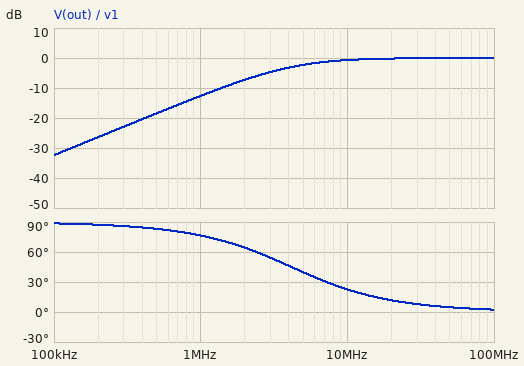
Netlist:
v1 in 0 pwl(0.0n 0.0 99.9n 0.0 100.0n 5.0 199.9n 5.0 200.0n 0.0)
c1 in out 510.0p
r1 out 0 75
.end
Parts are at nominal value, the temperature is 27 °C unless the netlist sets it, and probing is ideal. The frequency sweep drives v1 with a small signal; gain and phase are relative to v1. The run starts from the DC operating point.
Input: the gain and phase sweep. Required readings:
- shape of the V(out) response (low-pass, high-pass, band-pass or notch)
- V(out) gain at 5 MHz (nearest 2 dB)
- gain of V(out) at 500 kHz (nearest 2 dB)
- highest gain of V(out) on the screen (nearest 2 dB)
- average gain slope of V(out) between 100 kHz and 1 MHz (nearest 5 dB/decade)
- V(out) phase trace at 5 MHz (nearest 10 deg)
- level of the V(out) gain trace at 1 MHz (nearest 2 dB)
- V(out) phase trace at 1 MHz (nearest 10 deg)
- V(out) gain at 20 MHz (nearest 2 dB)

high-pass
-2 dB
-18 dB
0 dB
20 dB/decade
40 deg
-12 dB
80 deg
0 dB
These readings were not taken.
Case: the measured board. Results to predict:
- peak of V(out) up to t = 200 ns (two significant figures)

5.0 V
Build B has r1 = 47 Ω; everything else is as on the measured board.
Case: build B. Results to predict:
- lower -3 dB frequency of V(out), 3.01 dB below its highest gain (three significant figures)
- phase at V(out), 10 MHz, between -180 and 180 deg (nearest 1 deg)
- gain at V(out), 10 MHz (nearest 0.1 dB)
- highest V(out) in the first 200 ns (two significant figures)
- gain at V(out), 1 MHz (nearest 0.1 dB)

6.64 MHz
34 deg
-1.6 dB
5.0 V
-16.5 dB
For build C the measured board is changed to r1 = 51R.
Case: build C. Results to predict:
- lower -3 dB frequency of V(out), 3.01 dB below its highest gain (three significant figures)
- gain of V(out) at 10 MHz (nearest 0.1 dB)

6.12 MHz
-1.4 dB
